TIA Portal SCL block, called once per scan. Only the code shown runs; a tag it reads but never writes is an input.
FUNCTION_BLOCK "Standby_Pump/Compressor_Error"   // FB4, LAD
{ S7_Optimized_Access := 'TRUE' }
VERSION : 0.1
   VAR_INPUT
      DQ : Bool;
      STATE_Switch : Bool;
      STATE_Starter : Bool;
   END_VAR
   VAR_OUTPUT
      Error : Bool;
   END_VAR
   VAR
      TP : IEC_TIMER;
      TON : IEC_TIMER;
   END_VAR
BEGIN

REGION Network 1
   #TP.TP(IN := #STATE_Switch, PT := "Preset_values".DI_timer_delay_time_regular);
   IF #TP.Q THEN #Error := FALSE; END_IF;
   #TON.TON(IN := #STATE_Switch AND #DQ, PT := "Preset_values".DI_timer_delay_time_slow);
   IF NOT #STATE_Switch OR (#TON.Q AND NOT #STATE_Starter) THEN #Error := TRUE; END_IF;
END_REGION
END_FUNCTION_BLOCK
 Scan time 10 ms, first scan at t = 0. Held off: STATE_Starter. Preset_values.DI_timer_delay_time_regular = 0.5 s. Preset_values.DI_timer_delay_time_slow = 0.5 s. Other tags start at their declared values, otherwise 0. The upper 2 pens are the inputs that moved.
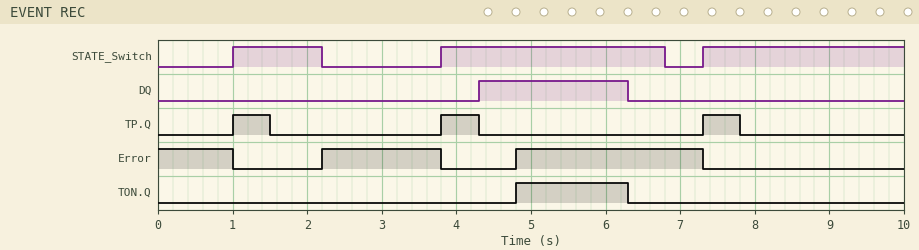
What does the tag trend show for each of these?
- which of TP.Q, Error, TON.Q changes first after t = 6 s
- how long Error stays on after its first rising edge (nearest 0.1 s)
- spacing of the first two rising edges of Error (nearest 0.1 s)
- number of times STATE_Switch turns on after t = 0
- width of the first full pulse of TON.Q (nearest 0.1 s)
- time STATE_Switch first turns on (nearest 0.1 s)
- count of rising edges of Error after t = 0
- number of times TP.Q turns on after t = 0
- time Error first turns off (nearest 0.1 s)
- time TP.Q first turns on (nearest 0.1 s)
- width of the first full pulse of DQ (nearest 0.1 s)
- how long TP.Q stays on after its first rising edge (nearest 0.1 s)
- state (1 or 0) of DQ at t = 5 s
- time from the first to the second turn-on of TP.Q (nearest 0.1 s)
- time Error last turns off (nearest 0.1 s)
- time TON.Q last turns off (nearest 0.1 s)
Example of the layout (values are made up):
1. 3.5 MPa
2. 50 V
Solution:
1. TON.Q
2. 1.6 s
3. 2.6 s
4. 3
5. 1.5 s
6. 1.0 s
7. 2
8. 3
9. 1.0 s
10. 1.0 s
11. 2.0 s
12. 0.5 s
13. 1
14. 2.8 s
15. 7.3 s
16. 6.3 s
